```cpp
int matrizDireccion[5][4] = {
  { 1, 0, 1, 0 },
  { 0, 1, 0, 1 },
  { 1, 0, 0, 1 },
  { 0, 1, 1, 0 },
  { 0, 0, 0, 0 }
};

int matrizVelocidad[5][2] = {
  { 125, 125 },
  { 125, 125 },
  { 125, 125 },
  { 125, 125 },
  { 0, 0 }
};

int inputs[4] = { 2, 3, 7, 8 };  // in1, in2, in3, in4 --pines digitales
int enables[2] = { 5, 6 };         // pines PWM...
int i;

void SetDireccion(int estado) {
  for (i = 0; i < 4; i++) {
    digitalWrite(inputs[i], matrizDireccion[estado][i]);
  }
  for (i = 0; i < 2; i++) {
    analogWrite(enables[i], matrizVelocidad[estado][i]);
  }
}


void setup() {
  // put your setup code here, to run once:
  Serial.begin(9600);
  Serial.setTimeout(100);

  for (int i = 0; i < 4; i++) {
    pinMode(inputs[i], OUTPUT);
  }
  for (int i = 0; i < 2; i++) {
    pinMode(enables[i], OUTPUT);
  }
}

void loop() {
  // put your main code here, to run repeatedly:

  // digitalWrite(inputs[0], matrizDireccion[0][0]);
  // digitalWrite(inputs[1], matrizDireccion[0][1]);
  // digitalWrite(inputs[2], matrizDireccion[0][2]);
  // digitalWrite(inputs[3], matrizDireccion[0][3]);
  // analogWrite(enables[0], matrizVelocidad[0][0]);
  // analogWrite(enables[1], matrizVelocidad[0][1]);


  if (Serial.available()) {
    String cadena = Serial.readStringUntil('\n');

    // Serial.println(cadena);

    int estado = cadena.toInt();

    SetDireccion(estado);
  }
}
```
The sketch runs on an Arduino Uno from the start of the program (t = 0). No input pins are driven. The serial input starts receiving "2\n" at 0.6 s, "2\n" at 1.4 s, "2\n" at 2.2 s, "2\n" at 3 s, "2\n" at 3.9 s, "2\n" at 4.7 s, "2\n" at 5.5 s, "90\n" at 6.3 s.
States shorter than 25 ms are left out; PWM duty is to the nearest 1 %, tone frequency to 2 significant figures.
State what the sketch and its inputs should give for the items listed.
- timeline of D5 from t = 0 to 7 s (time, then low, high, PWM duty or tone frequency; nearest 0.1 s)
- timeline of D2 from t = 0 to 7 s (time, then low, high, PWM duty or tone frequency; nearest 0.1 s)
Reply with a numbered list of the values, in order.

1. 0 s low; 0.6 s PWM 49 %; 6.3 s low
2. 0 s low; 0.6 s high; 6.3 s low
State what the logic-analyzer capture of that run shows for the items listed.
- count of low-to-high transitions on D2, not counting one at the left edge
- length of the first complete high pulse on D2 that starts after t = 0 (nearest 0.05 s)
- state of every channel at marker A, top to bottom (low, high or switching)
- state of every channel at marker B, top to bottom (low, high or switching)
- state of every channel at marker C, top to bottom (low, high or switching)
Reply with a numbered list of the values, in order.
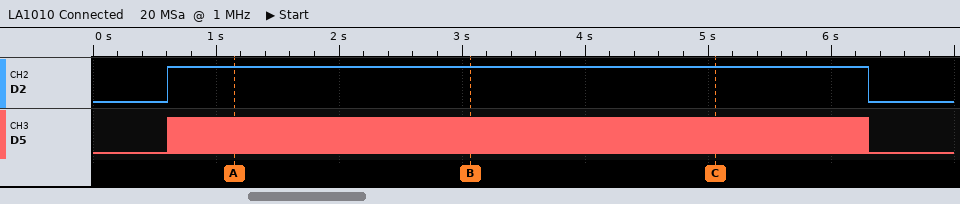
1. 1
2. 5.70 s
3. D2 high, D5 switching
4. D2 high, D5 switching
5. D2 high, D5 switching
